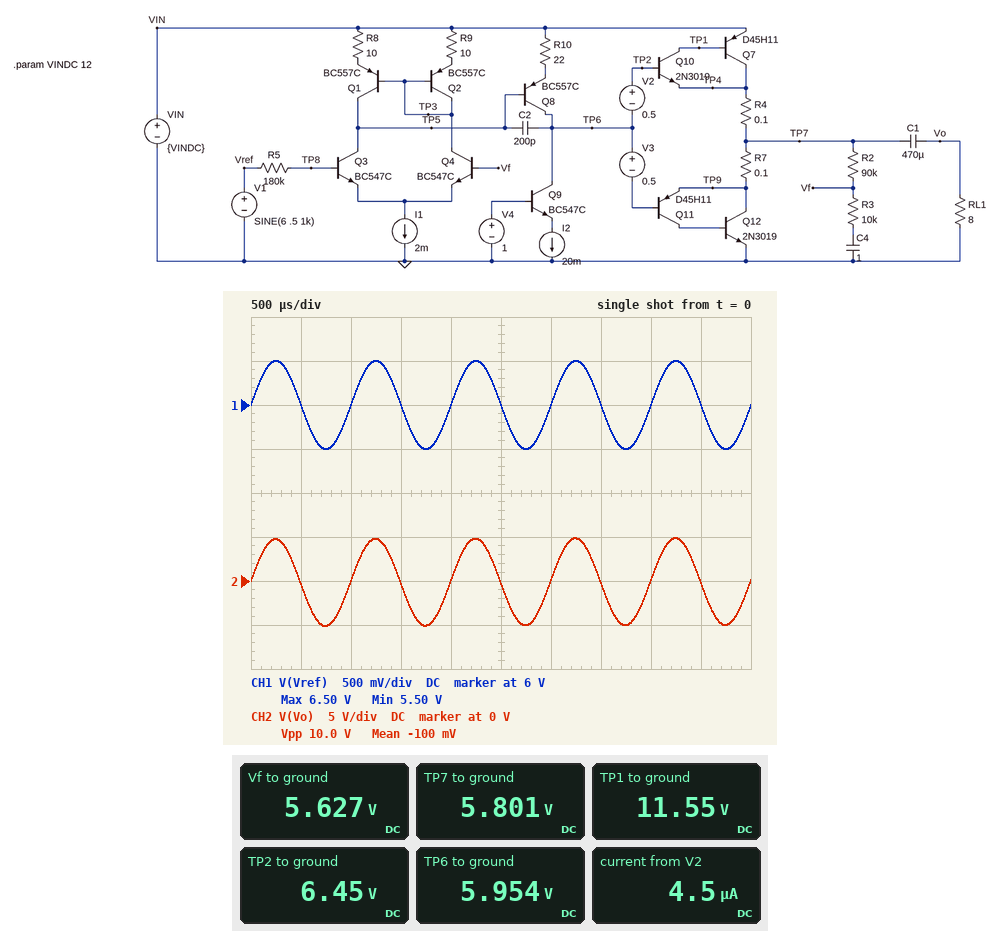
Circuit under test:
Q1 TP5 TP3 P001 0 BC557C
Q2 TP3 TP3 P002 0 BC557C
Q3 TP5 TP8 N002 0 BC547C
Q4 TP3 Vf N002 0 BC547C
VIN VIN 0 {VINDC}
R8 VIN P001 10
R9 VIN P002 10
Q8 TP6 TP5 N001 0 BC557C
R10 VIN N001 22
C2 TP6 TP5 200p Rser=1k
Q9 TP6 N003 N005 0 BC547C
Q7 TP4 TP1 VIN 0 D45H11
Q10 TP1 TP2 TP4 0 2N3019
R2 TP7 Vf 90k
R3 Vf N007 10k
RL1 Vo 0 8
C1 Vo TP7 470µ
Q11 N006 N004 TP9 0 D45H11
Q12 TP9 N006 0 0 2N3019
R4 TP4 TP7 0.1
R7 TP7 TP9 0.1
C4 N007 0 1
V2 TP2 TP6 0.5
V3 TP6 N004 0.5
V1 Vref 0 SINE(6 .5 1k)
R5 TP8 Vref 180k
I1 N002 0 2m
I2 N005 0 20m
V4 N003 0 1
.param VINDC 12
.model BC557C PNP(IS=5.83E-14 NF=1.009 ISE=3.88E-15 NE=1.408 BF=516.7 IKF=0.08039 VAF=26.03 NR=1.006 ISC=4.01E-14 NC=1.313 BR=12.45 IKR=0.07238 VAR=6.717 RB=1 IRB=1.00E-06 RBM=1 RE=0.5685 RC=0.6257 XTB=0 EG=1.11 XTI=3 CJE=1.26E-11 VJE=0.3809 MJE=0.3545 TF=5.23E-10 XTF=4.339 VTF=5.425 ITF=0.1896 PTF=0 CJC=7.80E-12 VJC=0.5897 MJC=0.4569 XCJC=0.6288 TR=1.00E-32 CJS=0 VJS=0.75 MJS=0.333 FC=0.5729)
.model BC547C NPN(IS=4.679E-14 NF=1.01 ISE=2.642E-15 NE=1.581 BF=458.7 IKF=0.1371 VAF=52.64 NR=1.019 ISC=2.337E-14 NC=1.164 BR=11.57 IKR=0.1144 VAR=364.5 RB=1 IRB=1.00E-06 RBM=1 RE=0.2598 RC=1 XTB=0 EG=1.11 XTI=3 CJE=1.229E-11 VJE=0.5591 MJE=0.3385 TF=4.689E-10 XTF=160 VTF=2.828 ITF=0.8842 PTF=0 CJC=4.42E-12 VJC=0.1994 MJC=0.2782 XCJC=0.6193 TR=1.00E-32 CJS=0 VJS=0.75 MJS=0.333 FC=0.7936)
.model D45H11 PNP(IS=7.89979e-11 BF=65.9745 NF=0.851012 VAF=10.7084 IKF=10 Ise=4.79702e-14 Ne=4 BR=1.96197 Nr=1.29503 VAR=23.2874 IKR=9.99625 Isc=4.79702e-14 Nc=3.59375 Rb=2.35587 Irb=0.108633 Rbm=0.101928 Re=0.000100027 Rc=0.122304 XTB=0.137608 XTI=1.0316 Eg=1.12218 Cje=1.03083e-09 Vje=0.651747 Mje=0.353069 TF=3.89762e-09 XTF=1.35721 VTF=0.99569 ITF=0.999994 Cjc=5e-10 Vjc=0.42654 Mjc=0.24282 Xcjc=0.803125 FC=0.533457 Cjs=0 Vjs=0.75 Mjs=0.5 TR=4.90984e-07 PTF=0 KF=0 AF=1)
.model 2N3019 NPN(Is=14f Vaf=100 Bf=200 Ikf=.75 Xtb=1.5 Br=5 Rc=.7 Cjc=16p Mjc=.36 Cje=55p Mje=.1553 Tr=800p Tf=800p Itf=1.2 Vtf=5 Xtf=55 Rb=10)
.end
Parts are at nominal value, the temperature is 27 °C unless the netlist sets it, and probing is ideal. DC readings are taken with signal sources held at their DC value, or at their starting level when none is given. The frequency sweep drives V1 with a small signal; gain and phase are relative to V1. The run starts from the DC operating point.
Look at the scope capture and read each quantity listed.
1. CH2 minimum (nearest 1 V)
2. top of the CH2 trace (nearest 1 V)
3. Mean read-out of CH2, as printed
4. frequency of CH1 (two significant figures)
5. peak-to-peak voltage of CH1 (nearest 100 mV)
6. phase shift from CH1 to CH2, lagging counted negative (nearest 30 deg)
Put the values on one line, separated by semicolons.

-5 V; 5 V; -100 mV; 1.0 kHz; 1.0 V; 0 deg
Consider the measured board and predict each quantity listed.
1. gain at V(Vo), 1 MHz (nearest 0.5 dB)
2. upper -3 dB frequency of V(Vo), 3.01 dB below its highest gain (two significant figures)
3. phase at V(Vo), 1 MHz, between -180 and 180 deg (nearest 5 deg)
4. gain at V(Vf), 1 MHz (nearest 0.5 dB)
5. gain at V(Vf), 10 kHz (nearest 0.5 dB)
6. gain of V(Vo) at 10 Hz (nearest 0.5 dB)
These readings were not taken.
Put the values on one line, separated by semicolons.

1.5 dB; 260 kHz; -125 deg; -20.0 dB; 0 dB; 7.0 dB
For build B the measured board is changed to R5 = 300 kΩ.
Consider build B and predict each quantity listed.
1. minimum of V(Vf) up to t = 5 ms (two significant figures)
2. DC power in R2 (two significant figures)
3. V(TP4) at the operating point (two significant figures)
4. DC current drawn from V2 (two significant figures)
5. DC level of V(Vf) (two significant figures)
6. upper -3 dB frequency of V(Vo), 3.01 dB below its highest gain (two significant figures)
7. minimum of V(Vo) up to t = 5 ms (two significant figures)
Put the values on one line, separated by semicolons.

4.9 V; 330 nW; 5.6 V; 4.4 µA; 5.4 V; 160 kHz; -5.0 V
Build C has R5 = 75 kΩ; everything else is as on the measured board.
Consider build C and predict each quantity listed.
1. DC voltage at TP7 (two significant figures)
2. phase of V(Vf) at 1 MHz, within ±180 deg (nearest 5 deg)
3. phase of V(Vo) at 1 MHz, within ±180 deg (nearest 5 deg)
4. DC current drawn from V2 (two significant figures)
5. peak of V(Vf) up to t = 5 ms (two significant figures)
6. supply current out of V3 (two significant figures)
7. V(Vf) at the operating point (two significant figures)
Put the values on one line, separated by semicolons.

6.0 V; -100 deg; -115 deg; 4.6 µA; 6.3 V; 5.3 µA; 5.8 V
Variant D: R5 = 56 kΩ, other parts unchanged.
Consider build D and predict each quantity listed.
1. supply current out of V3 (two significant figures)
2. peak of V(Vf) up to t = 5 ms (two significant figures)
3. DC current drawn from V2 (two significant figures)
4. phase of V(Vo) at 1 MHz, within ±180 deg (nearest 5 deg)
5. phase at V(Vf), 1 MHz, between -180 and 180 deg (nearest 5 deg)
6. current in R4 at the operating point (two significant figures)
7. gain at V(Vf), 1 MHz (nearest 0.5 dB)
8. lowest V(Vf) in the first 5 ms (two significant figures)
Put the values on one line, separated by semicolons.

5.3 µA; 6.4 V; 4.6 µA; -110 deg; -95 deg; 95 mA; -9.5 dB; 5.4 V
